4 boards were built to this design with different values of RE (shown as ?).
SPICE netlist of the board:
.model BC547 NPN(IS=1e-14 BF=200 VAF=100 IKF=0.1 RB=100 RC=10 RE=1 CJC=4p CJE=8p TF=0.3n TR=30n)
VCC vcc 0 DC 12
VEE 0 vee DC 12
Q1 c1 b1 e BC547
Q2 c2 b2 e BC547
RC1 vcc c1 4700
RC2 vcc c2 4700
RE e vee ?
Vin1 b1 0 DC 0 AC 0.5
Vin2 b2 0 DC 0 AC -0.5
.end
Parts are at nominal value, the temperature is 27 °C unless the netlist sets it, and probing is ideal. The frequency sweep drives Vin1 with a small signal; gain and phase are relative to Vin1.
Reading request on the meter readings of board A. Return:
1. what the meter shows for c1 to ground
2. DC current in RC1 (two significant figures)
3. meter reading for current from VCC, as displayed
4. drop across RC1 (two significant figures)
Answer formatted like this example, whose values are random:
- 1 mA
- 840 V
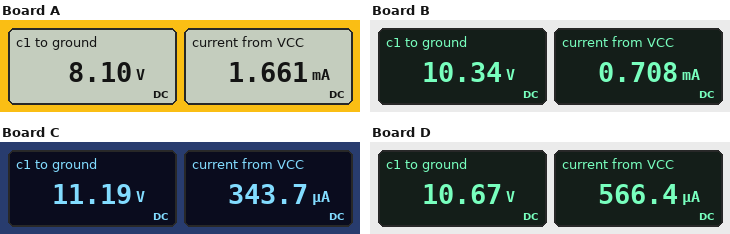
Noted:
- 8.10 V
- 830 µA
- 1.661 mA
- 3.9 V
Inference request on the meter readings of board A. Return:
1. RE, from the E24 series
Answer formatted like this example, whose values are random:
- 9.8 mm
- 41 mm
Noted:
- 6.8 kΩ
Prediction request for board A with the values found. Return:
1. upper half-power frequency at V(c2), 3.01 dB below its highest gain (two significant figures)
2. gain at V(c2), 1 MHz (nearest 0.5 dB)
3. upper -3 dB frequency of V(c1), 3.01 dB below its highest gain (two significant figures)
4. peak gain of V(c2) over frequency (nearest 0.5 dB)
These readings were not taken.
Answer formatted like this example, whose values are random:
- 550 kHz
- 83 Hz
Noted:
- 4.6 MHz
- 40.0 dB
- 4.6 MHz
- 40.5 dB
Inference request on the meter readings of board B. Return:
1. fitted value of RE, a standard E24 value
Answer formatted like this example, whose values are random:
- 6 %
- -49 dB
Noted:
- 16 kΩ
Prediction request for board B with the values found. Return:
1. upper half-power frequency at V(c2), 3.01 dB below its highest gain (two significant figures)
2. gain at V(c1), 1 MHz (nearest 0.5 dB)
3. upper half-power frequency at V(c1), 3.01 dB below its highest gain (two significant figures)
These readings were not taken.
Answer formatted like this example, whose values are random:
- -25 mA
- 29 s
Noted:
- 8.4 MHz
- 33.5 dB
- 8.4 MHz
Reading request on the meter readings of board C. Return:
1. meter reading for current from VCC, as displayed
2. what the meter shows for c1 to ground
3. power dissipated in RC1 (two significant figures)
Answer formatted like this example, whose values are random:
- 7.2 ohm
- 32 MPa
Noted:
- 343.7 µA
- 11.19 V
- 140 µW
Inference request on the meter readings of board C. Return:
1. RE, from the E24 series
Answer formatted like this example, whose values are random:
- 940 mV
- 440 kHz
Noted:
- 33 kΩ
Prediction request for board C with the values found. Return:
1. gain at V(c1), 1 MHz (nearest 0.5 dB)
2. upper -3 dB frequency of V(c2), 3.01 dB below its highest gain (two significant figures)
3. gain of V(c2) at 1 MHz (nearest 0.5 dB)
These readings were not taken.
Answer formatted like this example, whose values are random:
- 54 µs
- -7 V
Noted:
- 27.0 dB
- 12 MHz
- 27.0 dB
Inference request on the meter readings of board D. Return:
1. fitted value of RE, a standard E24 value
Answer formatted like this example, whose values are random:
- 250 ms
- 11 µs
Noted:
- 20 kΩ
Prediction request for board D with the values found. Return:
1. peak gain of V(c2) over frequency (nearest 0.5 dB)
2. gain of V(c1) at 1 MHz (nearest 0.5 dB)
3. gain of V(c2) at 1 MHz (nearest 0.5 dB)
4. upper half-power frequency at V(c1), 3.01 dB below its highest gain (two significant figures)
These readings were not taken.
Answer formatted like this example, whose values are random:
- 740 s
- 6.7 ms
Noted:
- 31.5 dB
- 31.5 dB
- 31.5 dB
- 9.5 MHz
